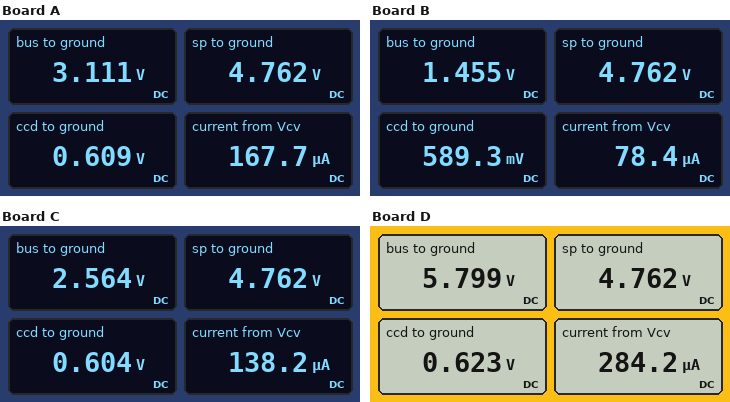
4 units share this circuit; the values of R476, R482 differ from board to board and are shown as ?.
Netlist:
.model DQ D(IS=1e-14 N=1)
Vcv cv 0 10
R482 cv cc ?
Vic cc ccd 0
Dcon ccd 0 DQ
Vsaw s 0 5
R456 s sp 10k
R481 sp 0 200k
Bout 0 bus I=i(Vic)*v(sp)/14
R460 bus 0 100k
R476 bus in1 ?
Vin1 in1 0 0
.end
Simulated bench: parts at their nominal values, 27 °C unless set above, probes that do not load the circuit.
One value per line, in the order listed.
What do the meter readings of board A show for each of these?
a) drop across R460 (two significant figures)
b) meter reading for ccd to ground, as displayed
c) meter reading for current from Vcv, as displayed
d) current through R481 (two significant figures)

3.1 V
0.609 V
167.7 µA
24 µA
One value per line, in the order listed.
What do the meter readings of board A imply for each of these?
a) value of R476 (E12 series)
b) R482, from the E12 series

120 kΩ
56 kΩ
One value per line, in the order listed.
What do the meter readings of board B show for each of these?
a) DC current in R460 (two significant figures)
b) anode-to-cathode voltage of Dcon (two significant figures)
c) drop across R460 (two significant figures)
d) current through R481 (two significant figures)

15 µA
590 mV
1.5 V
24 µA
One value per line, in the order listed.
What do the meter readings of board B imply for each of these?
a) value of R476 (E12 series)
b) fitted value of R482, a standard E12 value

120 kΩ
120 kΩ
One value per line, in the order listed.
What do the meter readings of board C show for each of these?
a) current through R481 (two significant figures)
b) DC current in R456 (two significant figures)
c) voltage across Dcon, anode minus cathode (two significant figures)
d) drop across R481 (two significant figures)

24 µA
24 µA
600 mV
4.8 V
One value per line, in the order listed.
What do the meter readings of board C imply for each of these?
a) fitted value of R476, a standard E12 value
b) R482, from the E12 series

120 kΩ
68 kΩ
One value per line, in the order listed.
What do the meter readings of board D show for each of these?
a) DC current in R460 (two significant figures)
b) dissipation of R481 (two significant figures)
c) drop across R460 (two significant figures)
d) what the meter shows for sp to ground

58 µA
110 µW
5.8 V
4.762 V
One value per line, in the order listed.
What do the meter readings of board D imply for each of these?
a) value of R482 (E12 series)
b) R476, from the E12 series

33 kΩ
150 kΩ
